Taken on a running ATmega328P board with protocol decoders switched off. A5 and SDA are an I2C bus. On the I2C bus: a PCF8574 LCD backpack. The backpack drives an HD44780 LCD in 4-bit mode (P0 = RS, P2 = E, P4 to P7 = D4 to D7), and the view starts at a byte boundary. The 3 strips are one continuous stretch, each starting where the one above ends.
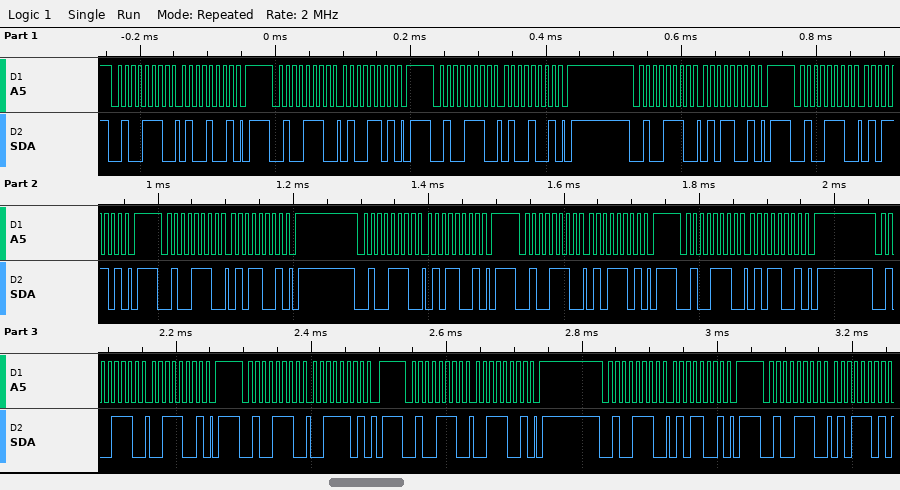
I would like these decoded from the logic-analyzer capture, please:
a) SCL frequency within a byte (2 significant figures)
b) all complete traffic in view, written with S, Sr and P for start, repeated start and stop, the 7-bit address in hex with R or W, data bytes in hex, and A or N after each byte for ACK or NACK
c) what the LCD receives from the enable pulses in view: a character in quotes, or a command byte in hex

100 kHz
S 27W A 49 A P S 27W A 4D A P S 27W A 49 A P S 27W A 59 A P S 27W A 5D A P S 27W A 59 A P S 27W A 59 A P S 27W A 5D A P S 27W A 59 A P S 27W A 39 A P S 27W A 3D A P S 27W A 39 A P S 27W A 59 A P S 27W A 5D A
'E' 'S'
